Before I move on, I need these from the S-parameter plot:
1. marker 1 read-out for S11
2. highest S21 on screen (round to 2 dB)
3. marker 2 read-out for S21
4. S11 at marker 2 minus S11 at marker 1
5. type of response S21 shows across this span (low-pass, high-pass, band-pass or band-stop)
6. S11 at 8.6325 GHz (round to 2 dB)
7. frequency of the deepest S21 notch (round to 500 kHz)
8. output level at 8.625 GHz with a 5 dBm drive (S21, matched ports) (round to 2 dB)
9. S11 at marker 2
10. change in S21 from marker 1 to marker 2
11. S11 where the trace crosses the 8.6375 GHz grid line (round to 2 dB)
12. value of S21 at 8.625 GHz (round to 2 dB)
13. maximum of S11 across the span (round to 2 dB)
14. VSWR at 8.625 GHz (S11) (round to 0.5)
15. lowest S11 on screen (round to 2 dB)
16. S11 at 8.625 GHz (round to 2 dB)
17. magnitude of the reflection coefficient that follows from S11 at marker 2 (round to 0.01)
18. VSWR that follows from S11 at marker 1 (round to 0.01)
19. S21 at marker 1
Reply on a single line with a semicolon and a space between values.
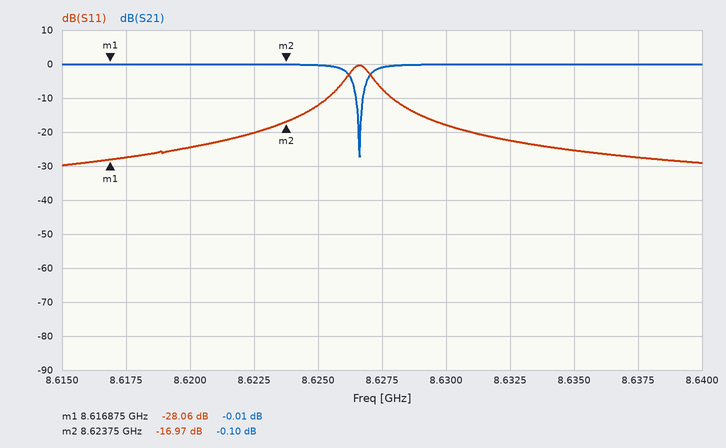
-28.06 dB; 0 dB; -0.10 dB; 11.09 dB; band-stop; -22 dB; 8.6265 GHz; 4 dBm; -16.97 dB; -0.09 dB; -28 dB; 0 dB; 0 dB; 1.5; -30 dB; -12 dB; 0.14; 1.08; -0.01 dB
